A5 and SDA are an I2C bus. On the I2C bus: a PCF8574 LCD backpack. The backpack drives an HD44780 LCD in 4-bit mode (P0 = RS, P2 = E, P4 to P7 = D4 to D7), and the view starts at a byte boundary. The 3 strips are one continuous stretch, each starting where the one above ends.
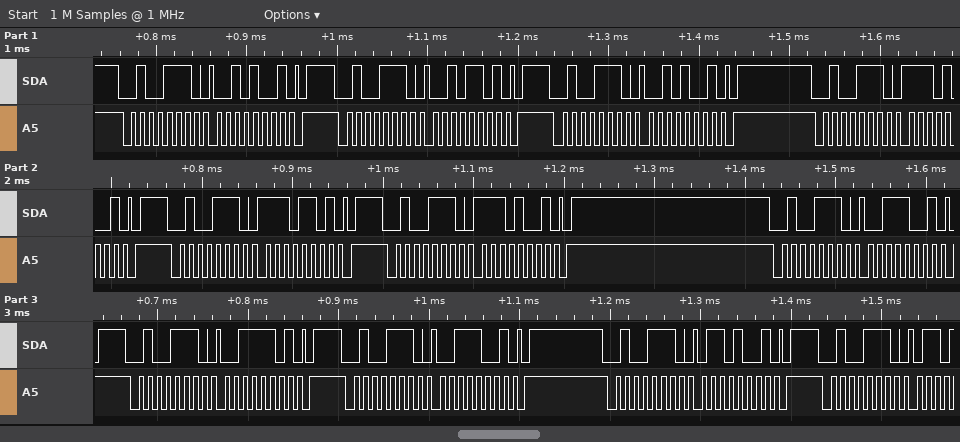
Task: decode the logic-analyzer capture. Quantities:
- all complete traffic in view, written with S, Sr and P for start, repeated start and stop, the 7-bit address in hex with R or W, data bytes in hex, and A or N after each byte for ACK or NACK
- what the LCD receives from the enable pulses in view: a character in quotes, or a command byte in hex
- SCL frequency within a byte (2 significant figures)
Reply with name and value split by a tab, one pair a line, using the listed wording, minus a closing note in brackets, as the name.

all complete traffic in view, written with S, Sr and P for start, repeated start and stop, the 7-bit address in hex with R or W, data bytes in hex, and A or N after each byte for ACK or NACK	S 27W A 29 A P S 27W A 2D A P S 27W A 29 A P S 27W A E9 A P S 27W A ED A P S 27W A E9 A P S 27W A 39 A P S 27W A 3D A P S 27W A 39 A P S 27W A 69 A P S 27W A
what the LCD receives from the enable pulses in view: a character in quotes, or a command byte in hex	'.'
SCL frequency within a byte	100 kHz
